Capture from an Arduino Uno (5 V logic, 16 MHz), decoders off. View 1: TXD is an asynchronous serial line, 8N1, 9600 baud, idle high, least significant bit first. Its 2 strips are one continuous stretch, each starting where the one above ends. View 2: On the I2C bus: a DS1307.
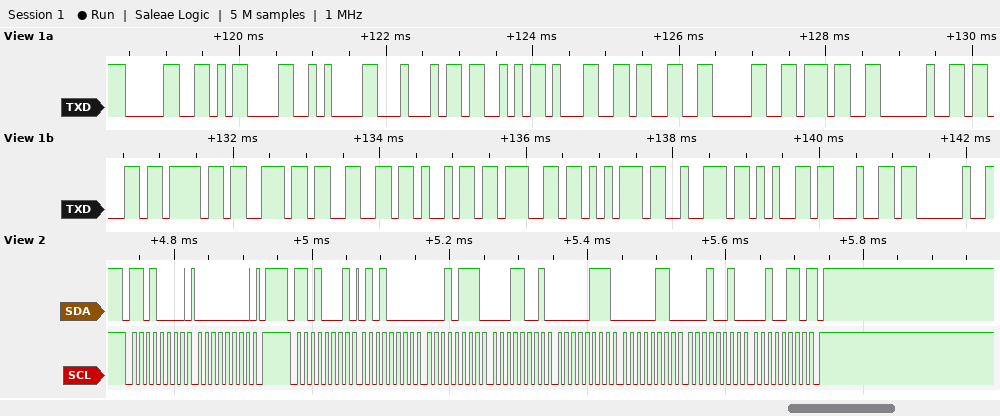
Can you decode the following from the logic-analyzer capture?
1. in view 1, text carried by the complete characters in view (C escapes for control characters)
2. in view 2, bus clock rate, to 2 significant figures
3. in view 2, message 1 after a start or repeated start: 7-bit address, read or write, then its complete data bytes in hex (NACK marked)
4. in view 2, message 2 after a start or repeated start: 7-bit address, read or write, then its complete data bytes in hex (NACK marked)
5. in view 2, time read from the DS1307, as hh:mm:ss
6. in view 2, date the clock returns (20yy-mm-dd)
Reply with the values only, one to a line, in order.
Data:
"0\r\nDS1307 configured "
100 kHz
0x68 write: 00
0x68 read: 50 17 19 07 06 12 26 NACK
19:17:50
2026-12-06
